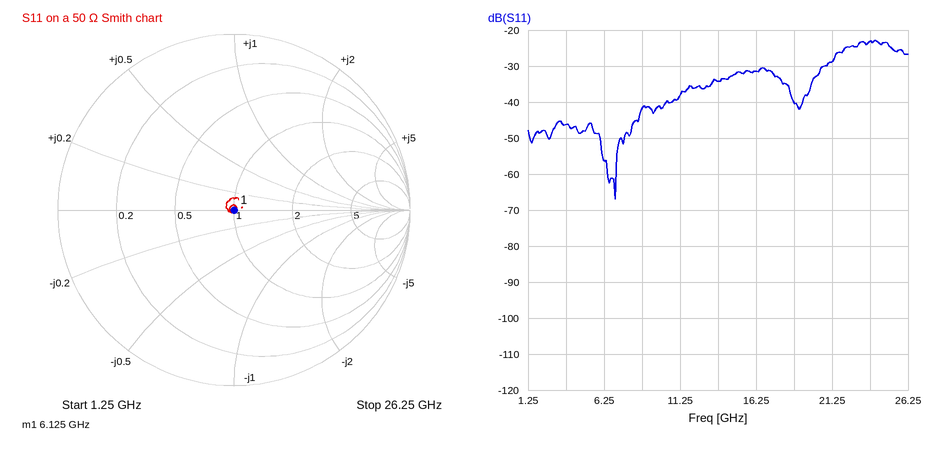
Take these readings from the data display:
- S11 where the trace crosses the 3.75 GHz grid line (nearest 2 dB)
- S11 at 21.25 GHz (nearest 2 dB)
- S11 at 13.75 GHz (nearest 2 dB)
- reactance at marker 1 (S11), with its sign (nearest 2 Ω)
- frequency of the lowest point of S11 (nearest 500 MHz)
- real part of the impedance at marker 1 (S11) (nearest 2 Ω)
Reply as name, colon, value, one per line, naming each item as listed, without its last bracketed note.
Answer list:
S11 where the trace crosses the 3.75 GHz grid line: -46 dB
S11 at 21.25 GHz: -28 dB
S11 at 13.75 GHz: -34 dB
reactance at marker 1 (S11), with its sign: 0 Ω
frequency of the lowest point of S11: 7.0 GHz
real part of the impedance at marker 1 (S11): 50 Ω
